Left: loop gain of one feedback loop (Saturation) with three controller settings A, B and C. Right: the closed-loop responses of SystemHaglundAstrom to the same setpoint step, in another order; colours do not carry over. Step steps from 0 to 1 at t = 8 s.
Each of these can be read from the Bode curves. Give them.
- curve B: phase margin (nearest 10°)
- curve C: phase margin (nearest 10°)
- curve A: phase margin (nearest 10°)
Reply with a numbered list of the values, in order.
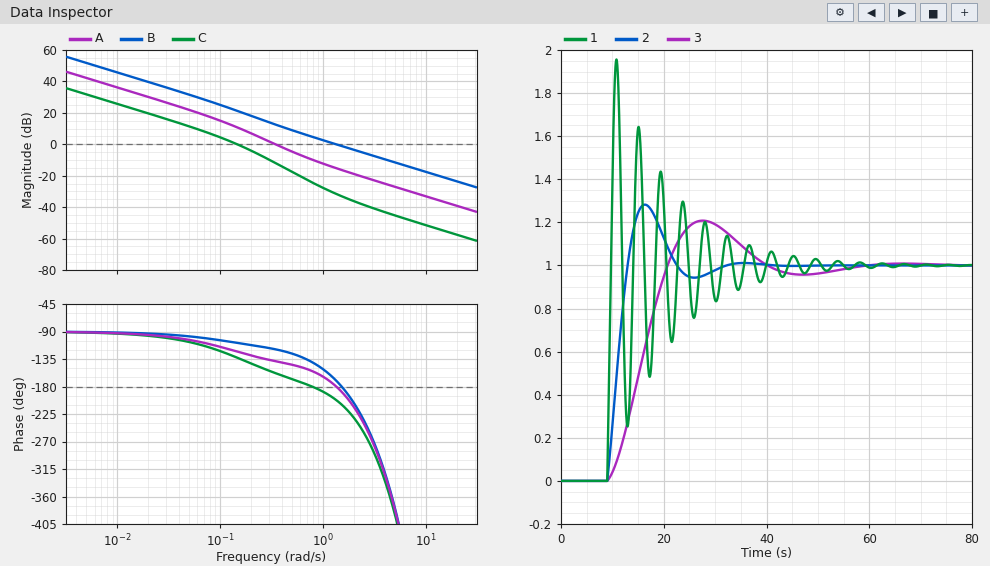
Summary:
1. 10°
2. 50°
3. 40°
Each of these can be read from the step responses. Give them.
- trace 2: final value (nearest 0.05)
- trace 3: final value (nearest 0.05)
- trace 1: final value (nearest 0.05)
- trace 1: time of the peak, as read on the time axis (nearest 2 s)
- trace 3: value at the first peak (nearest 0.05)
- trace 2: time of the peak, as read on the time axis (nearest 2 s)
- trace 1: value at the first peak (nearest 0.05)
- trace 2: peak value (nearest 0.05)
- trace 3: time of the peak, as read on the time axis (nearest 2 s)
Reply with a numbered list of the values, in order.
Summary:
1. 1.00
2. 1.00
3. 1.00
4. 10 s
5. 1.20
6. 16 s
7. 1.95
8. 1.30
9. 28 s
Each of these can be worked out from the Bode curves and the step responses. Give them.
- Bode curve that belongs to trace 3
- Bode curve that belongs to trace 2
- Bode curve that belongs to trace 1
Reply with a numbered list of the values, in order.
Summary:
1. C
2. A
3. B
